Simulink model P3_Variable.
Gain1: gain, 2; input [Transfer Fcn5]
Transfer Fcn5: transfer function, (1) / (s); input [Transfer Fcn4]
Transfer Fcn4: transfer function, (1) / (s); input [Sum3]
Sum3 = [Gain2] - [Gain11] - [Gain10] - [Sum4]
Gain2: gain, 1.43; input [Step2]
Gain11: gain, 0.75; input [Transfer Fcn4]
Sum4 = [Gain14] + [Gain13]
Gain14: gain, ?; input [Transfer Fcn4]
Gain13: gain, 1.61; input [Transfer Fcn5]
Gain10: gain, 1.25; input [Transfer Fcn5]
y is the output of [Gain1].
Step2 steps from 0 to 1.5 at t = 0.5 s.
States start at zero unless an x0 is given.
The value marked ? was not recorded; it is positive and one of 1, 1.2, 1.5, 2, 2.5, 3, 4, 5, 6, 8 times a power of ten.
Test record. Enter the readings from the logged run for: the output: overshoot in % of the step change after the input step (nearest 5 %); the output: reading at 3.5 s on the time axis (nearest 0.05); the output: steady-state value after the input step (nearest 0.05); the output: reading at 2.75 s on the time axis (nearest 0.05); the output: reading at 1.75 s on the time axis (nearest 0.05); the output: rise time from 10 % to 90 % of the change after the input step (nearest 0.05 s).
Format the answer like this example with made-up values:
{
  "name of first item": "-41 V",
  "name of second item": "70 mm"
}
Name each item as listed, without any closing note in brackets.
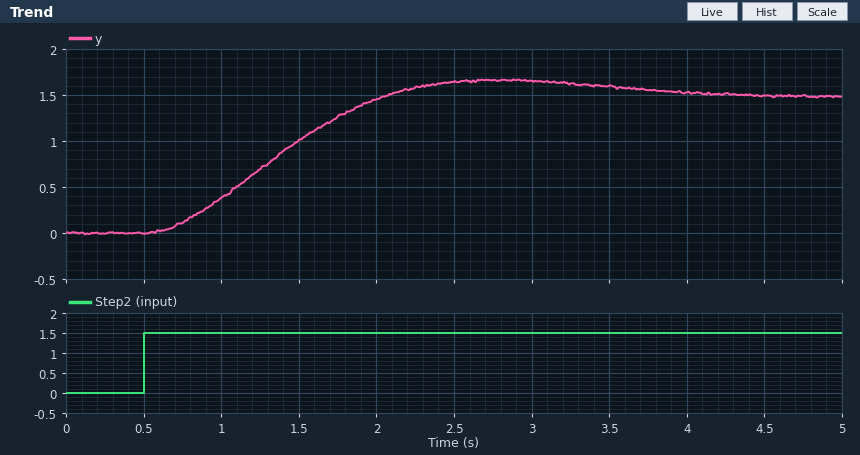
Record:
{
  "the output: overshoot in % of the step change after the input step": "10 %",
  "the output: reading at 3.5 s on the time axis": "1.60",
  "the output: steady-state value after the input step": "1.50",
  "the output: reading at 2.75 s on the time axis": "1.65",
  "the output: reading at 1.75 s on the time axis": "1.25",
  "the output: rise time from 10 % to 90 % of the change after the input step": "1.05 s"
}
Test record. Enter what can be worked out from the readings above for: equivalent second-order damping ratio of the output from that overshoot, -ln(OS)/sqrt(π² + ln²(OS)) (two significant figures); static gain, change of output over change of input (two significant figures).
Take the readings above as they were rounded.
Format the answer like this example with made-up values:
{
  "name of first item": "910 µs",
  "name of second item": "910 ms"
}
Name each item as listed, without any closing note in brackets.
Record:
{
  "equivalent second-order damping ratio of the output from that overshoot, -ln(OS)/sqrt(π² + ln²(OS))": "0.59",
  "static gain, change of output over change of input": "1.0"
}
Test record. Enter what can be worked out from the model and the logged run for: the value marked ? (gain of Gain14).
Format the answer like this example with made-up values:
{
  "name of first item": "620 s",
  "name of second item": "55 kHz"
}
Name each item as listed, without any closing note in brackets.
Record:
{
  "the value marked ?": "1.2"
}
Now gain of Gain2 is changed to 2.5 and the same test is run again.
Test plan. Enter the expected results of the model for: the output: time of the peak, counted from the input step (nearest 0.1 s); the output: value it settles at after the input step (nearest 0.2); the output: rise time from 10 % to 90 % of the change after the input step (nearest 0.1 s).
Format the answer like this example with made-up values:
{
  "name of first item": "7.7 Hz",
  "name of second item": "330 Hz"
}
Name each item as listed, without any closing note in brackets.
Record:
{
  "the output: time of the peak, counted from the input step": "2.3 s",
  "the output: value it settles at after the input step": "2.6",
  "the output: rise time from 10 % to 90 % of the change after the input step": "1.1 s"
}
